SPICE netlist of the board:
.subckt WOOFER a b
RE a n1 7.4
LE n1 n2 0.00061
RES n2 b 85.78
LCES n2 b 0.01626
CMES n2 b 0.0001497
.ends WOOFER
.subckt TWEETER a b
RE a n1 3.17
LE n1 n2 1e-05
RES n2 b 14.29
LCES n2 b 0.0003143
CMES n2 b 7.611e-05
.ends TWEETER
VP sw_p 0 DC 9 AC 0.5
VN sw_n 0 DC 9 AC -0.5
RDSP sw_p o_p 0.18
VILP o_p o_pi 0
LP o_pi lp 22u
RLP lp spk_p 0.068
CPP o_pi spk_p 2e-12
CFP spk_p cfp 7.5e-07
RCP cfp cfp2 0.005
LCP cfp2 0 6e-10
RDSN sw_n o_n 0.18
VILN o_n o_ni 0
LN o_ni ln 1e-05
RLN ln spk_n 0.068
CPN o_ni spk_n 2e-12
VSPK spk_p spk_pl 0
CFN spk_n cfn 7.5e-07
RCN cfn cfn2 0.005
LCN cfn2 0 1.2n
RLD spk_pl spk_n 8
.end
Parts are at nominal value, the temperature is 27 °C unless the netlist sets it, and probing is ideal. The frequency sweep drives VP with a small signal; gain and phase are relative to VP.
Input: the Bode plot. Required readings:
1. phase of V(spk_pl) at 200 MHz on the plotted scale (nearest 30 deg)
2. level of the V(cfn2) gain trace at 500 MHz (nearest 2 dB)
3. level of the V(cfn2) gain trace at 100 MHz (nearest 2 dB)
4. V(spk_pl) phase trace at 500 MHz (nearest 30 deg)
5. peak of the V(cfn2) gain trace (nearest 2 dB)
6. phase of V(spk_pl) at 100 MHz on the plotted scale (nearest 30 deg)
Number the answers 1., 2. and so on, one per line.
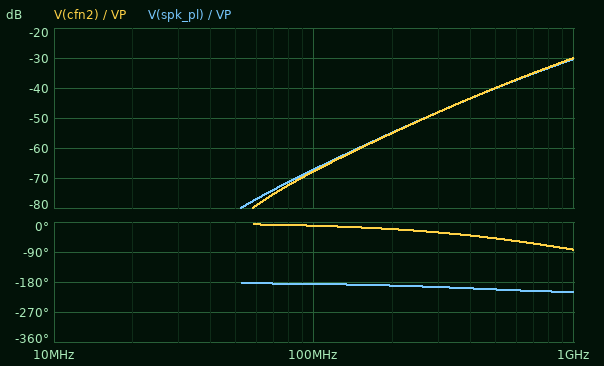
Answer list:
1. -180 deg
2. -40 dB
3. -68 dB
4. -210 deg
5. -30 dB
6. -180 deg
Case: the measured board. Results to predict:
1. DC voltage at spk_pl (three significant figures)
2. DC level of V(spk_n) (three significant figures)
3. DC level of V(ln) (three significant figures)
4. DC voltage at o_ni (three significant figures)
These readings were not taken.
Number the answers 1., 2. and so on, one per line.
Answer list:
1. 9.00 V
2. 9.00 V
3. 9.00 V
4. 9.00 V
